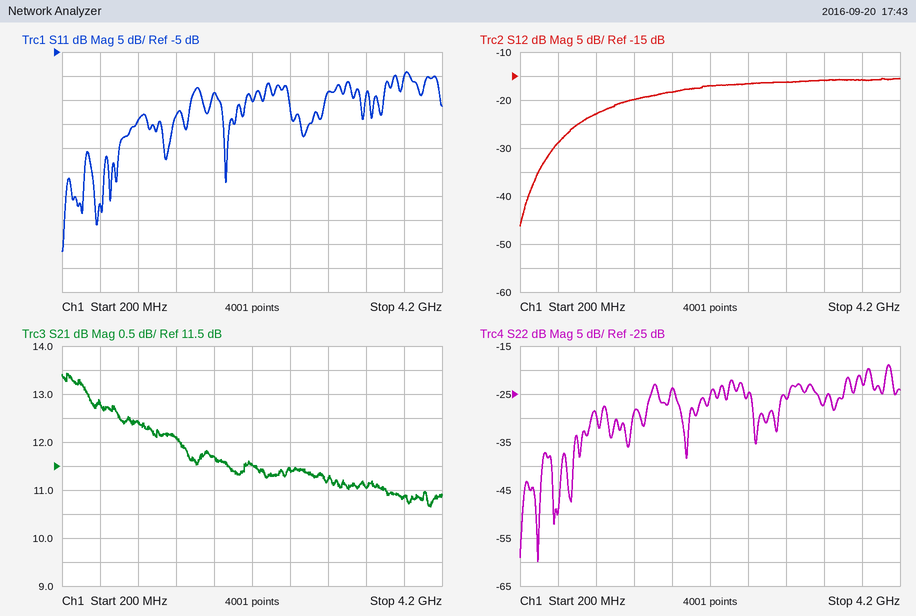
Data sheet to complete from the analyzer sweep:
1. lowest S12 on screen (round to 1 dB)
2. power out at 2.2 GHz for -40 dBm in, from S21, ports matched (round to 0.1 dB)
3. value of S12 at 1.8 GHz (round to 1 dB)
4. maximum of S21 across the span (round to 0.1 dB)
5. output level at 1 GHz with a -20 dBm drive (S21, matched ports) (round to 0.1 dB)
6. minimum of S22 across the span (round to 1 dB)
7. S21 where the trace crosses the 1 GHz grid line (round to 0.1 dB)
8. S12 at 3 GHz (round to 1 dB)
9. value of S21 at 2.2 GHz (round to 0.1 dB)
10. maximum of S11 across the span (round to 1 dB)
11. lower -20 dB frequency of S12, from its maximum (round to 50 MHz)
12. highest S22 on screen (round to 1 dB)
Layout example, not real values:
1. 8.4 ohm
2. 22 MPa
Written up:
1. -46 dB
2. -28.5 dBm
3. -18 dB
4. 13.4 dB
5. -7.6 dBm
6. -60 dB
7. 12.4 dB
8. -16 dB
9. 11.5 dB
10. -9 dB
11. 400 MHz
12. -19 dB
